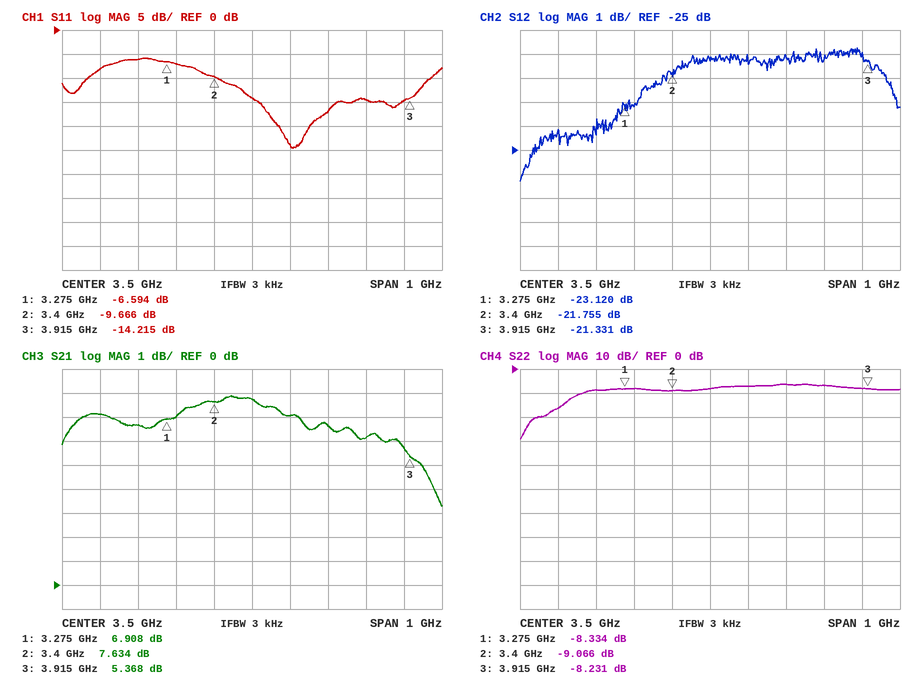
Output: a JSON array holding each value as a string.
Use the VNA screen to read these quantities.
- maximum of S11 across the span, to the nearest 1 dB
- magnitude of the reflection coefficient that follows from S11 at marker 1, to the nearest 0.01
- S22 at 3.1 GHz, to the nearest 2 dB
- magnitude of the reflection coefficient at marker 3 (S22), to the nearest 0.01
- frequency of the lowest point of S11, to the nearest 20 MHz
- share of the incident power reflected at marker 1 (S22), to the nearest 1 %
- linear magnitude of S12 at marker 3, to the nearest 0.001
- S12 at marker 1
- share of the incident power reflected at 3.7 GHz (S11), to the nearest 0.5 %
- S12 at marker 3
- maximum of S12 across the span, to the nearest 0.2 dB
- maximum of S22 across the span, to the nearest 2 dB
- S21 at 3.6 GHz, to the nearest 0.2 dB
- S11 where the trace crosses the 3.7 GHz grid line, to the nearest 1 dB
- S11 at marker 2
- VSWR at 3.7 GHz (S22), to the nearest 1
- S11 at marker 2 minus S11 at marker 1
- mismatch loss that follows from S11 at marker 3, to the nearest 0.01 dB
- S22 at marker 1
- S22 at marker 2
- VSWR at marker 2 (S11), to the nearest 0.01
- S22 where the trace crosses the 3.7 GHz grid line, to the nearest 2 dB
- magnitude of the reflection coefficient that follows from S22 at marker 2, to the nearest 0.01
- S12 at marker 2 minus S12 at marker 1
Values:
["-6 dB", "0.47", "-16 dB", "0.39", "3.60 GHz", "15 %", "0.086", "-23.120 dB", "2.0 %", "-21.331 dB", "-20.8 dB", "-6 dB", "7.0 dB", "-17 dB", "-9.666 dB", "3", "-3.072 dB", "0.17 dB", "-8.334 dB", "-9.066 dB", "1.98", "-6 dB", "0.35", "1.365 dB"]
